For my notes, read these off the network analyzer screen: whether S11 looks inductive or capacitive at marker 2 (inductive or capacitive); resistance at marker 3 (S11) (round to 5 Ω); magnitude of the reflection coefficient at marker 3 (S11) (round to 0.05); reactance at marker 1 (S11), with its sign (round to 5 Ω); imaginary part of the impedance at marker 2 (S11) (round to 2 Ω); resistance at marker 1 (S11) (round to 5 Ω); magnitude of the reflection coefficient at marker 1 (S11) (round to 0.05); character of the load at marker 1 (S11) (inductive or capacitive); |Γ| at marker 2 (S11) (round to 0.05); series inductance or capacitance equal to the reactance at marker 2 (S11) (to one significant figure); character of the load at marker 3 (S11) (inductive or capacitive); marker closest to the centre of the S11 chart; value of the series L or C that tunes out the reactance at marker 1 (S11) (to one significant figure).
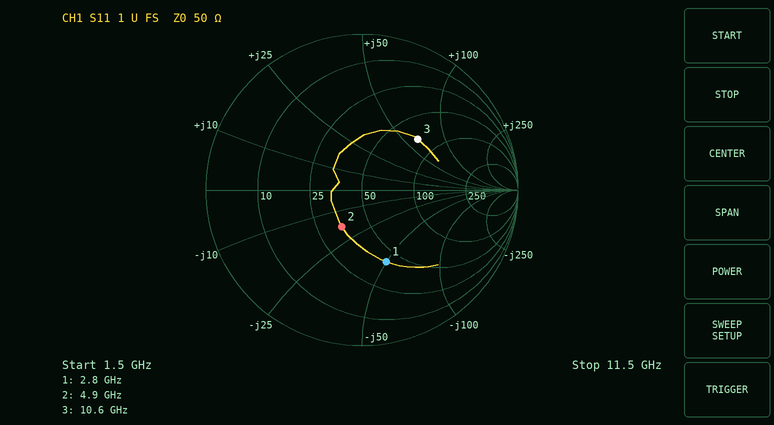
capacitive
75 Ω
0.50
-50 Ω
-18 Ω
40 Ω
0.50
capacitive
0.25
2 pF
inductive
marker 2
3 nH
